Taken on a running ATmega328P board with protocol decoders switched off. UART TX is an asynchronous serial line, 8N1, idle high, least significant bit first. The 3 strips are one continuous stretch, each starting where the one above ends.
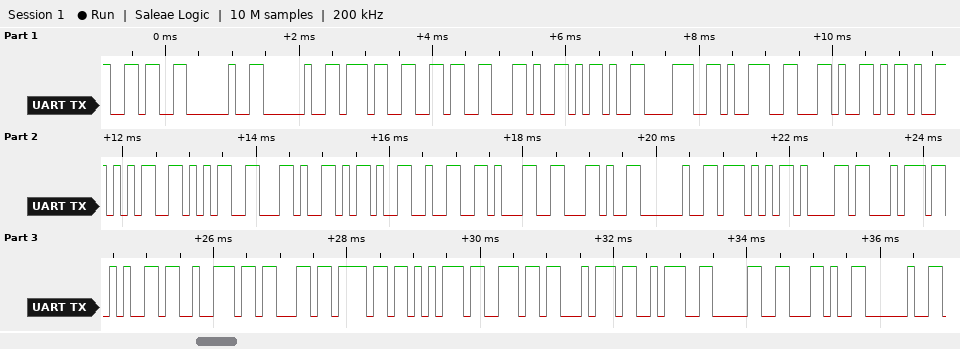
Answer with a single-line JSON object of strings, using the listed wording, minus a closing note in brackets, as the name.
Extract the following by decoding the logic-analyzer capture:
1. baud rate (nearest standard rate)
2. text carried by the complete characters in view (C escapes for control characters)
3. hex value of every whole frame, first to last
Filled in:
{"baud rate": "9600 baud", "text carried by the complete characters in view": "\"6  76,-89,-55,-21, Watercount:0, \"", "hex value of every whole frame, first to last": "0x36 0x20 0x20 0x37 0x36 0x2C 0x2D 0x38 0x39 0x2C 0x2D 0x35 0x35 0x2C 0x2D 0x32 0x31 0x2C 0x20 0x57 0x61 0x74 0x65 0x72 0x63 0x6F 0x75 0x6E 0x74 0x3A 0x30 0x2C 0x20"}
